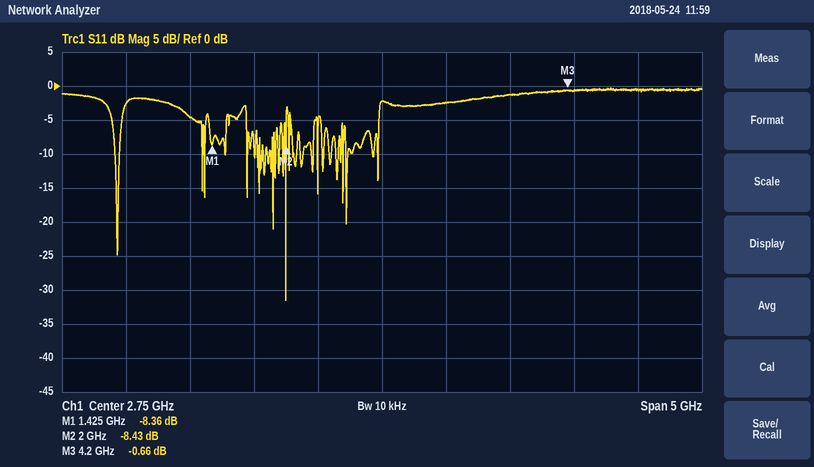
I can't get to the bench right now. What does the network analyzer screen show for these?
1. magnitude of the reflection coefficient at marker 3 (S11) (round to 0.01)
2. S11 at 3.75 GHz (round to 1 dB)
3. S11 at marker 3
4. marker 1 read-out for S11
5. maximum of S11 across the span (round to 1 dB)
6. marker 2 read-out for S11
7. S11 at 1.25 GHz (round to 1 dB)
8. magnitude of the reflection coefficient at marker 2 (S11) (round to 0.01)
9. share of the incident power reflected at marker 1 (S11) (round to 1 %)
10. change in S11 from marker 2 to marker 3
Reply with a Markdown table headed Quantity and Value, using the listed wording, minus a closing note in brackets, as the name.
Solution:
| Quantity | Value |
|---|---|
| magnitude of the reflection coefficient at marker 3 (S11) | 0.93 |
| S11 at 3.75 GHz | -1 dB |
| S11 at marker 3 | -0.66 dB |
| marker 1 read-out for S11 | -8.36 dB |
| maximum of S11 across the span | 0 dB |
| marker 2 read-out for S11 | -8.43 dB |
| S11 at 1.25 GHz | -5 dB |
| magnitude of the reflection coefficient at marker 2 (S11) | 0.38 |
| share of the incident power reflected at marker 1 (S11) | 15 % |
| change in S11 from marker 2 to marker 3 | 7.77 dB |
